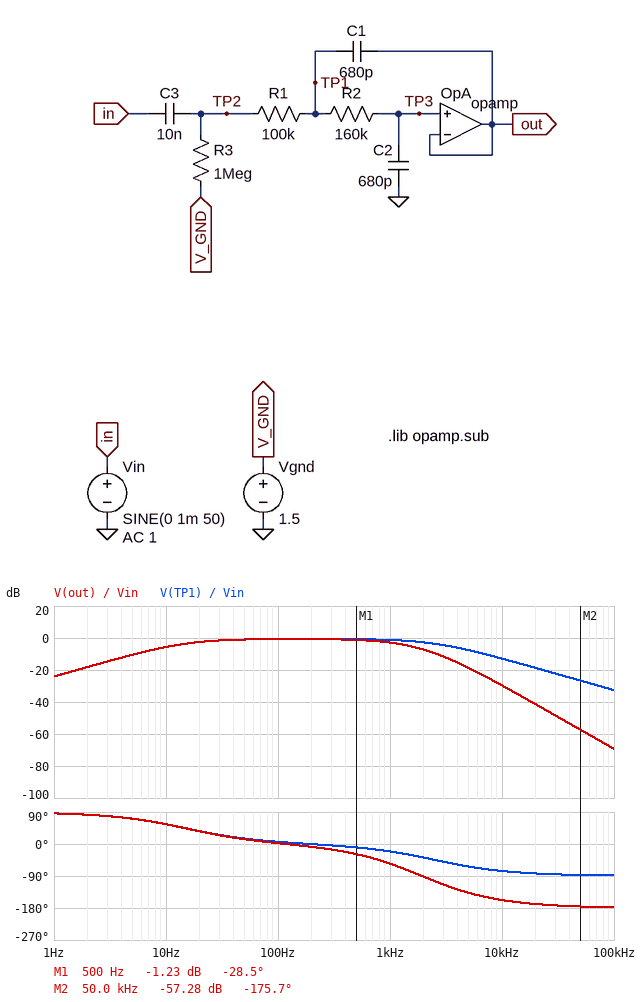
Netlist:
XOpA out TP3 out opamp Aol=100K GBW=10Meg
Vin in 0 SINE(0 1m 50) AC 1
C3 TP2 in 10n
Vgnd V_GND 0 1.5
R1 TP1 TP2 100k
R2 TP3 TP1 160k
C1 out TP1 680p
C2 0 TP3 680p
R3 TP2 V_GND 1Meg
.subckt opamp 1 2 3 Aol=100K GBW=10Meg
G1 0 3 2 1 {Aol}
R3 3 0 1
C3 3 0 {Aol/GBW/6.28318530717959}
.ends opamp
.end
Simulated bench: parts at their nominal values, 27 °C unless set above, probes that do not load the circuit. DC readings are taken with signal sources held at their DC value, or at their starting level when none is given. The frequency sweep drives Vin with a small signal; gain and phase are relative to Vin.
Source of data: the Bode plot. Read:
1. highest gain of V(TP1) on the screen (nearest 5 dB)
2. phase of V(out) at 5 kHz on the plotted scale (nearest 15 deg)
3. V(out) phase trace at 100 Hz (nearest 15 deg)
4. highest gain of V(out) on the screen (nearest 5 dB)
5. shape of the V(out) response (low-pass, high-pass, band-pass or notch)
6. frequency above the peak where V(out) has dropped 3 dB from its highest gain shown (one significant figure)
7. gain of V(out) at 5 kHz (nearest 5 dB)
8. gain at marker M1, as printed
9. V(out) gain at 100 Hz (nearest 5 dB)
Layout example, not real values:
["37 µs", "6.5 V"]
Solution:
["0 dB", "-135 deg", "0 deg", "0 dB", "band-pass", "1 kHz", "-20 dB", "-1.23 dB", "0 dB"]
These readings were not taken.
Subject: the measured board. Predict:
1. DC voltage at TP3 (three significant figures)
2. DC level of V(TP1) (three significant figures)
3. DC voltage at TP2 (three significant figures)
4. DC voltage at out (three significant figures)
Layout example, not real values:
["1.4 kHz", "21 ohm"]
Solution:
["1.50 V", "1.50 V", "1.50 V", "1.50 V"]
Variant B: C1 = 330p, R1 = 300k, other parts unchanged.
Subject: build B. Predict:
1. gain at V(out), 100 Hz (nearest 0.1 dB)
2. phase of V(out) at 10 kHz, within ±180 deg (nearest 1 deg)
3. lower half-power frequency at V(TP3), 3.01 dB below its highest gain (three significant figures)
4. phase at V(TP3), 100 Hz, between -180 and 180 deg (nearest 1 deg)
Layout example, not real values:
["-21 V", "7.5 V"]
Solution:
["-0.8 dB", "-154 deg", "14.2 Hz", "-2 deg"]
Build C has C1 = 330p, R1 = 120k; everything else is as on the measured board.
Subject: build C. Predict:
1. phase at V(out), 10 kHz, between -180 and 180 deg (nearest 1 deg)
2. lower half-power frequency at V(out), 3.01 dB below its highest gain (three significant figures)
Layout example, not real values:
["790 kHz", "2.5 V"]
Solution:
["-143 deg", "14.5 Hz"]
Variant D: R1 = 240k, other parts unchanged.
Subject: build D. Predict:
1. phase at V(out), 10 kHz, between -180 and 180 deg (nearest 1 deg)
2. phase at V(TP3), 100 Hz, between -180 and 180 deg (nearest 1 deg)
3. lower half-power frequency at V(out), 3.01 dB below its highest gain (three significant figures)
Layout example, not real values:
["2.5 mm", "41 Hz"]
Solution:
["-166 deg", "-1 deg", "14.4 Hz"]
